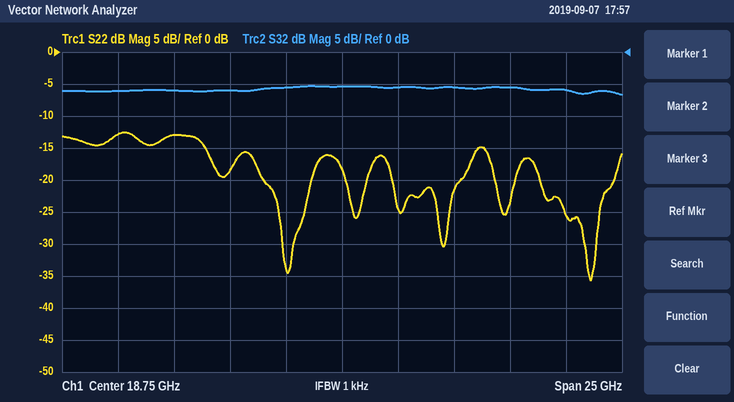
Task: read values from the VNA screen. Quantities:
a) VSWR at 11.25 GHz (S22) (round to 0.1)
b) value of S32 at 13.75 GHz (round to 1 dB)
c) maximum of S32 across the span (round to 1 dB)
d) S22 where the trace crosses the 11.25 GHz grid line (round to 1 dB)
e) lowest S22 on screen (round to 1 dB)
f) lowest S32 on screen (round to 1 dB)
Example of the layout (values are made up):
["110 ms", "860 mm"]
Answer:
["1.6", "-6 dB", "-5 dB", "-13 dB", "-36 dB", "-7 dB"]
